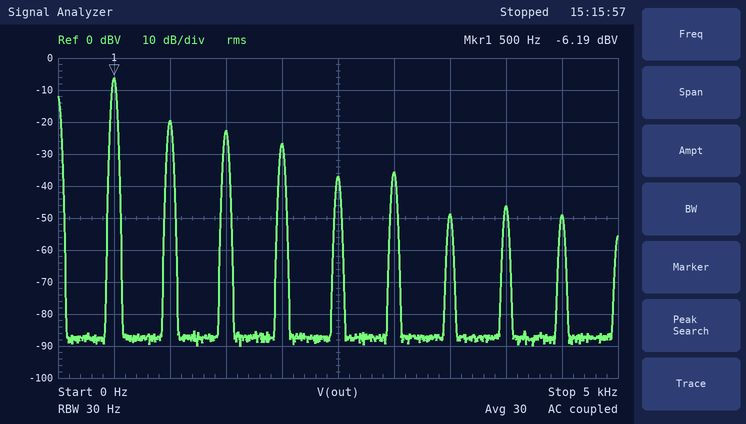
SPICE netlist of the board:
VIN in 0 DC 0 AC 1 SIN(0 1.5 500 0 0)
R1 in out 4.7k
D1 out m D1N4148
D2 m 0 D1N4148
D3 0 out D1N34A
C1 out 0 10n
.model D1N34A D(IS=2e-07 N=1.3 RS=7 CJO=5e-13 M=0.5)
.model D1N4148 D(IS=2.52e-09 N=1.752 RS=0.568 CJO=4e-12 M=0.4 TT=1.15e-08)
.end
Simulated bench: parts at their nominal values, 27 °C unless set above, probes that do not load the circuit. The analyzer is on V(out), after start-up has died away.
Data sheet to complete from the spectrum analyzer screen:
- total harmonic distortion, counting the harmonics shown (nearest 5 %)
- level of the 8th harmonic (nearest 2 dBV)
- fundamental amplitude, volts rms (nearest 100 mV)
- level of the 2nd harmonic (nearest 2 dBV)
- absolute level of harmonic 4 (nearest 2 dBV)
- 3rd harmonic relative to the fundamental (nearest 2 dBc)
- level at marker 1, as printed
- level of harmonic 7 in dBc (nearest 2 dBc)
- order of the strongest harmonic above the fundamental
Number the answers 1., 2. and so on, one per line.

1. 30 %
2. -46 dBV
3. 500 mV
4. -20 dBV
5. -26 dBV
6. -16 dBc
7. -6.19 dBV
8. -42 dBc
9. 2
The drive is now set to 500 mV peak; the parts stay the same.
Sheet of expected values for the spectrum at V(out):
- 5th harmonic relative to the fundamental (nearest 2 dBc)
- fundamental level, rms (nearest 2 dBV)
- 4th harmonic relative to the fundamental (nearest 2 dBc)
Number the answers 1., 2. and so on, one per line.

1. -36 dBc
2. -12 dBV
3. -36 dBc
